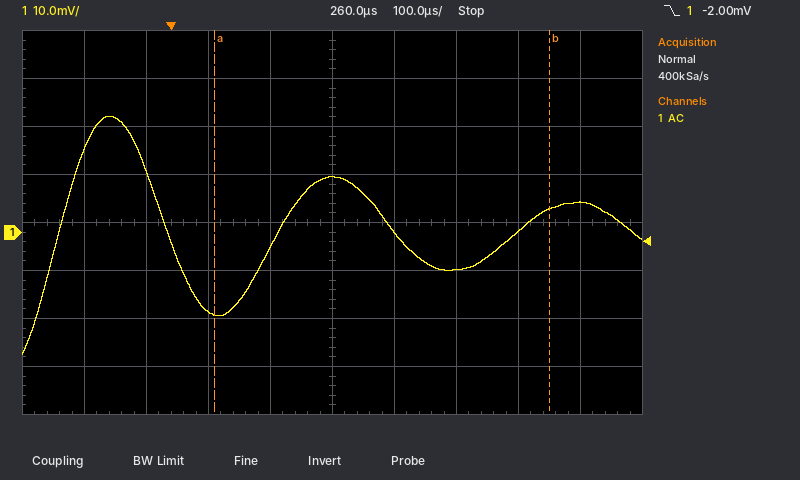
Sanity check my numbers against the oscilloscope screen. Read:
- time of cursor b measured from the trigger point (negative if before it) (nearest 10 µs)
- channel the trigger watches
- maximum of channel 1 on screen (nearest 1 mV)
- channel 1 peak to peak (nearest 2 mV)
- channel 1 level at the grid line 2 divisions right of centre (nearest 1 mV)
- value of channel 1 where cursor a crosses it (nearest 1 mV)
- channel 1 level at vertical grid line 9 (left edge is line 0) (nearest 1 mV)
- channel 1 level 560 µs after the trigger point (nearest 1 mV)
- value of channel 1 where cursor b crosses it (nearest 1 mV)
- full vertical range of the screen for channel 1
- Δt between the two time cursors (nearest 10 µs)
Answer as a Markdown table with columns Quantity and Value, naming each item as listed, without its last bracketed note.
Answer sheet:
| Quantity | Value |
|---|---|
| time of cursor b measured from the trigger point (negative if before it) | +610 µs |
| channel the trigger watches | channel 1 |
| maximum of channel 1 on screen | 24 mV |
| channel 1 peak to peak | 50 mV |
| channel 1 level at the grid line 2 divisions right of centre | -8 mV |
| value of channel 1 where cursor a crosses it | -17 mV |
| channel 1 level at vertical grid line 9 (left edge is line 0) | 6 mV |
| channel 1 level 560 µs after the trigger point | 0 mV |
| value of channel 1 where cursor b crosses it | 5 mV |
| full vertical range of the screen for channel 1 | 80 mV |
| Δt between the two time cursors | 540 µs |
